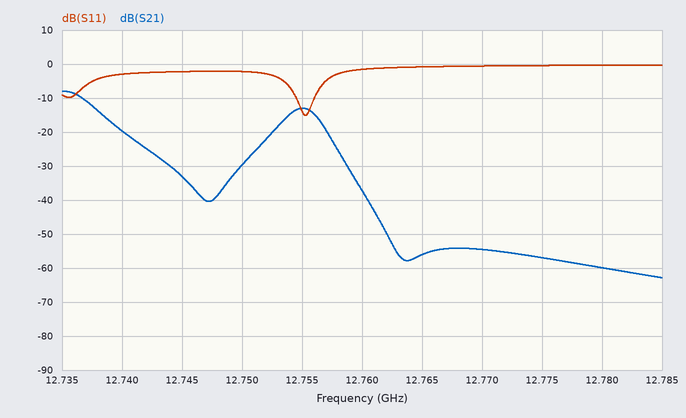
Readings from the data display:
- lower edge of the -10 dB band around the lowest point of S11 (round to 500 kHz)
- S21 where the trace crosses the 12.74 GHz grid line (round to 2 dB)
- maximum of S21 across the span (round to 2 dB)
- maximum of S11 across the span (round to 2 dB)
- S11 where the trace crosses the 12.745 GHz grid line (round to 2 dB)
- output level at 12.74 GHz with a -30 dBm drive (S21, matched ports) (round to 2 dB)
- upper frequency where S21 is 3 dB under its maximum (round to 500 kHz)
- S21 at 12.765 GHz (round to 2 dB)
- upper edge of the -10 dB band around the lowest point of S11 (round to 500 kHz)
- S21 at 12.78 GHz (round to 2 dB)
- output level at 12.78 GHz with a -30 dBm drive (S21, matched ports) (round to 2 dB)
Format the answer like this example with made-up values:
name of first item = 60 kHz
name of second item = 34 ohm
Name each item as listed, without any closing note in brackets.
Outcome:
lower edge of the -10 dB band around the lowest point of S11 = 12.7545 GHz
S21 where the trace crosses the 12.74 GHz grid line = -20 dB
maximum of S21 across the span = -8 dB
maximum of S11 across the span = 0 dB
S11 where the trace crosses the 12.745 GHz grid line = -2 dB
output level at 12.74 GHz with a -30 dBm drive (S21, matched ports) = -50 dBm
upper frequency where S21 is 3 dB under its maximum = 12.7370 GHz
S21 at 12.765 GHz = -56 dB
upper edge of the -10 dB band around the lowest point of S11 = 12.7560 GHz
S21 at 12.78 GHz = -60 dB
output level at 12.78 GHz with a -30 dBm drive (S21, matched ports) = -90 dBm
